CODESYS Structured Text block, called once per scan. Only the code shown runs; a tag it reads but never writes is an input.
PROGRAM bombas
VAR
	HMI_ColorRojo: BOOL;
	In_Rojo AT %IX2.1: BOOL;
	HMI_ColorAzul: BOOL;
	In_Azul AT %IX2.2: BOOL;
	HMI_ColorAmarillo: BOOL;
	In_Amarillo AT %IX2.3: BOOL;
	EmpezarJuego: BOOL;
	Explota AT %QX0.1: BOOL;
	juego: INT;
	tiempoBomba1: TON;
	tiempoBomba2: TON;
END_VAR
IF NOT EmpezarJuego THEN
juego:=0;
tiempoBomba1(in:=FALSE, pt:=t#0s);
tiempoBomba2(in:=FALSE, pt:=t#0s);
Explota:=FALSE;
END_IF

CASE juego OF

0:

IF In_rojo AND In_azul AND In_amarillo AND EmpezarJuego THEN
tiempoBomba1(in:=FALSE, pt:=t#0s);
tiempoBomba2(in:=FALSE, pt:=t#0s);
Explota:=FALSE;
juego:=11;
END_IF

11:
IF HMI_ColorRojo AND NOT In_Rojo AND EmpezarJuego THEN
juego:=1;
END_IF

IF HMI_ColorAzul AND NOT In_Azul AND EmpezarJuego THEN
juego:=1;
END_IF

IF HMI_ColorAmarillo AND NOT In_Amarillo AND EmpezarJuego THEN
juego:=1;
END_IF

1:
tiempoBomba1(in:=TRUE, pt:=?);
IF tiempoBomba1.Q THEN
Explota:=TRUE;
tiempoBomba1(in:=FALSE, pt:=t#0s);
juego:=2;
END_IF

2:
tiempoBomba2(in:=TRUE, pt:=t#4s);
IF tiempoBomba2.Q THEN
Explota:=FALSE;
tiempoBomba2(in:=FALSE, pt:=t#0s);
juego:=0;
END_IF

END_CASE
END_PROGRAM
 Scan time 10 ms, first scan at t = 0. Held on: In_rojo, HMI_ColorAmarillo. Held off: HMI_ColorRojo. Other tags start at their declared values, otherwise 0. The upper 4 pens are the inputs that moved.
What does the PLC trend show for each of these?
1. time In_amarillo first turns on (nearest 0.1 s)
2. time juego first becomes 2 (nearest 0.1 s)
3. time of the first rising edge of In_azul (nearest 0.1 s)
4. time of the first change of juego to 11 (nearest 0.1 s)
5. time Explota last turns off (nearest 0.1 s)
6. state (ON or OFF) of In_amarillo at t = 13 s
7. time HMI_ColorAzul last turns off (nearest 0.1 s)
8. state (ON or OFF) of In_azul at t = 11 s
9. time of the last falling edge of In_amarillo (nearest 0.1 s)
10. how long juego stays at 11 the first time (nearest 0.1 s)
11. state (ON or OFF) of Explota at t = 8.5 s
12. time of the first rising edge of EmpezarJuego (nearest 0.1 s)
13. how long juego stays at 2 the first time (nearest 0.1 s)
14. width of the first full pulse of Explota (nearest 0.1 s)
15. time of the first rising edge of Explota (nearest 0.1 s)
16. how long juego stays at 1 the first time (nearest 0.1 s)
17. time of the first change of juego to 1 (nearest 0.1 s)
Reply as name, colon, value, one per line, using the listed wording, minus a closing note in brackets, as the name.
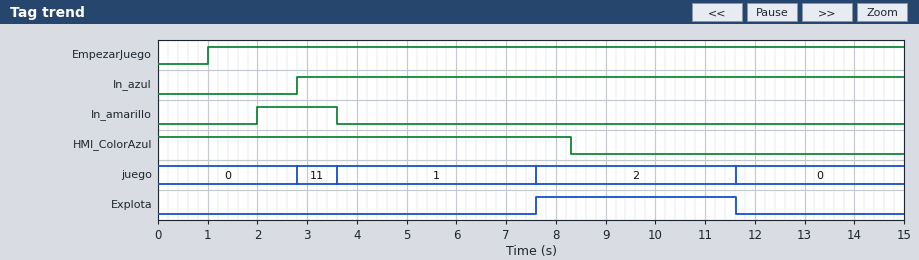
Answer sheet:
time In_amarillo first turns on: 2.0 s
time juego first becomes 2: 7.6 s
time of the first rising edge of In_azul: 2.8 s
time of the first change of juego to 11: 2.8 s
time Explota last turns off: 11.6 s
state (ON or OFF) of In_amarillo at t = 13 s: OFF
time HMI_ColorAzul last turns off: 8.3 s
state (ON or OFF) of In_azul at t = 11 s: ON
time of the last falling edge of In_amarillo: 3.6 s
how long juego stays at 11 the first time: 0.8 s
state (ON or OFF) of Explota at t = 8.5 s: ON
time of the first rising edge of EmpezarJuego: 1.0 s
how long juego stays at 2 the first time: 4.0 s
width of the first full pulse of Explota: 4.0 s
time of the first rising edge of Explota: 7.6 s
how long juego stays at 1 the first time: 4.0 s
time of the first change of juego to 1: 3.6 s
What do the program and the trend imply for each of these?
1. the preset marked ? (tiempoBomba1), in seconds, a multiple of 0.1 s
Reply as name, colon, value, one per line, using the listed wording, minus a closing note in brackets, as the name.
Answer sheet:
the preset marked ? (tiempoBomba1), in seconds, a multiple of 0.1 s: 4.0 s
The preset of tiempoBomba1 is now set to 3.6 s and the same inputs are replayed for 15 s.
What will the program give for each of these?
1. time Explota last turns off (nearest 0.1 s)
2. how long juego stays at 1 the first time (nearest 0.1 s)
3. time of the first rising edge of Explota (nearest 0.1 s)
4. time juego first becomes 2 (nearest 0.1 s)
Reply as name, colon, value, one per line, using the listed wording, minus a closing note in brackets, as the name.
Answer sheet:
time Explota last turns off: 11.2 s
how long juego stays at 1 the first time: 3.6 s
time of the first rising edge of Explota: 7.2 s
time juego first becomes 2: 7.2 s
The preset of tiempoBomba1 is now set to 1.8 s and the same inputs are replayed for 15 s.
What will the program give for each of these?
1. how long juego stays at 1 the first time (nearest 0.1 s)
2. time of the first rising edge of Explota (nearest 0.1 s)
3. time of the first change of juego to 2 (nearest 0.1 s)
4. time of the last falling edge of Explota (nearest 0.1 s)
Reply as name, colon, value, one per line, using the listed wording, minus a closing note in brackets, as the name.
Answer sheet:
how long juego stays at 1 the first time: 1.8 s
time of the first rising edge of Explota: 5.4 s
time of the first change of juego to 2: 5.4 s
time of the last falling edge of Explota: 9.4 s
